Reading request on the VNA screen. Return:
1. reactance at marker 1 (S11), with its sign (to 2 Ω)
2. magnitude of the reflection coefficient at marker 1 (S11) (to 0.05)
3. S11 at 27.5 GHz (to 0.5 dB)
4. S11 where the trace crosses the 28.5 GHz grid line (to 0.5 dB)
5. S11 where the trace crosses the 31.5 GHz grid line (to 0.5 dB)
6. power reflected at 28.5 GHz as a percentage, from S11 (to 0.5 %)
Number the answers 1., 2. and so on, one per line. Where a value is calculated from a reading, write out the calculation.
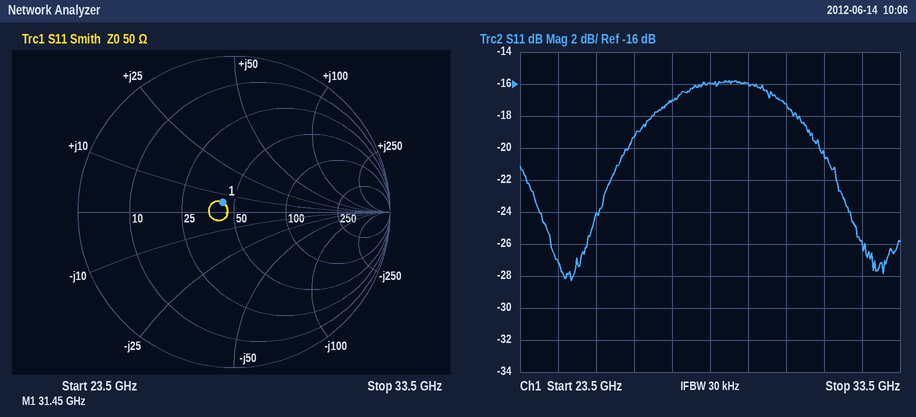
1. +6 Ω
2. 0.10
3. -17.0 dB
4. -16.0 dB
5. -20.5 dB
6. 10^(-16/10) ≈ 2.5 %
